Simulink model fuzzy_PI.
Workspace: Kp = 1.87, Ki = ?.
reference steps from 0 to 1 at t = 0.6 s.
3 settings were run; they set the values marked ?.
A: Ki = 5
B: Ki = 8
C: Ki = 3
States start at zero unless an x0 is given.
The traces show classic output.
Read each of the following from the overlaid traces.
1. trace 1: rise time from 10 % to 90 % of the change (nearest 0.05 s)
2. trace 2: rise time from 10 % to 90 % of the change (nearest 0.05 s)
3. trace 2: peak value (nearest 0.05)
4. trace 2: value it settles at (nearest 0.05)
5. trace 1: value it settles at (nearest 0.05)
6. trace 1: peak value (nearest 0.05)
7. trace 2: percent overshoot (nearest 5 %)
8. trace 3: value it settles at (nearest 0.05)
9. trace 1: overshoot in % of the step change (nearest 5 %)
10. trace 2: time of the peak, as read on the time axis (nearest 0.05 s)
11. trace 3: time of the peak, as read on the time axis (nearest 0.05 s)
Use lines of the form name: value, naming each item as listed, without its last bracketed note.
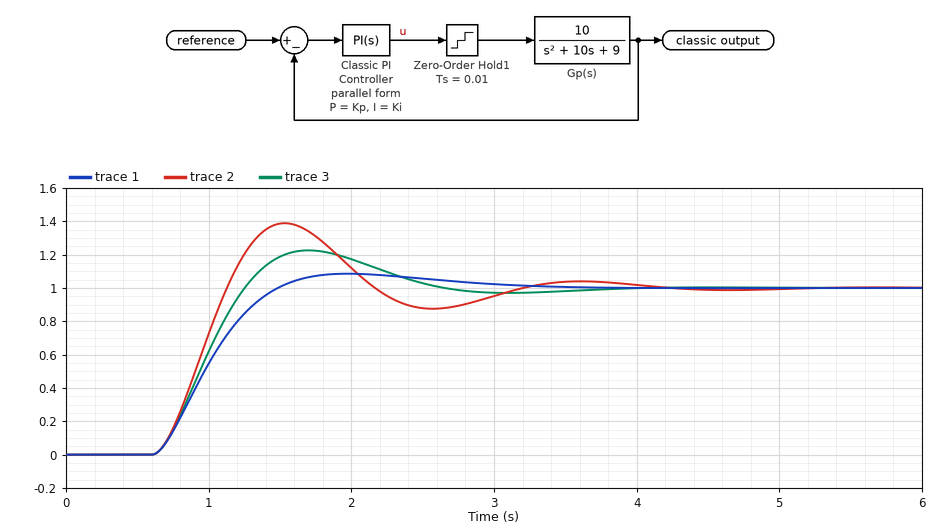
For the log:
trace 1: rise time from 10 % to 90 % of the change: 0.60 s
trace 2: rise time from 10 % to 90 % of the change: 0.35 s
trace 2: peak value: 1.40
trace 2: value it settles at: 1.00
trace 1: value it settles at: 1.00
trace 1: peak value: 1.10
trace 2: percent overshoot: 40 %
trace 3: value it settles at: 1.00
trace 1: overshoot in % of the step change: 10 %
trace 2: time of the peak, as read on the time axis: 1.55 s
trace 3: time of the peak, as read on the time axis: 1.70 s
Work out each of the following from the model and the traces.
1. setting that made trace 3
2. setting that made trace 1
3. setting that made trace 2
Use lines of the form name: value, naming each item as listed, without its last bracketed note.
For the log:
setting that made trace 3: A
setting that made trace 1: C
setting that made trace 2: B
